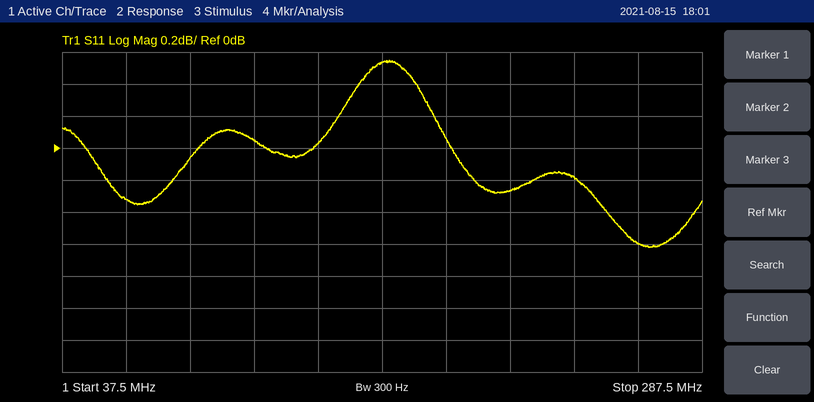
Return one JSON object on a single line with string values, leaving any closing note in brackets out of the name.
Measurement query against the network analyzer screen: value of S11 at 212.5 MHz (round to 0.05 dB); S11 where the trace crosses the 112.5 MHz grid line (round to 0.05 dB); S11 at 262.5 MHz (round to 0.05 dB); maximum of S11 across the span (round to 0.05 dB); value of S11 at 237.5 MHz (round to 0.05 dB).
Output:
{"value of S11 at 212.5 MHz": "-0.25 dB", "S11 where the trace crosses the 112.5 MHz grid line": "0.05 dB", "S11 at 262.5 MHz": "-0.60 dB", "maximum of S11 across the span": "0.55 dB", "value of S11 at 237.5 MHz": "-0.20 dB"}
